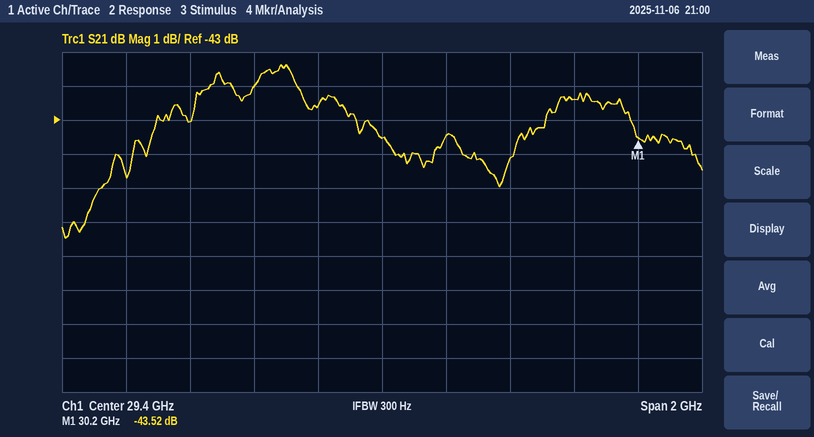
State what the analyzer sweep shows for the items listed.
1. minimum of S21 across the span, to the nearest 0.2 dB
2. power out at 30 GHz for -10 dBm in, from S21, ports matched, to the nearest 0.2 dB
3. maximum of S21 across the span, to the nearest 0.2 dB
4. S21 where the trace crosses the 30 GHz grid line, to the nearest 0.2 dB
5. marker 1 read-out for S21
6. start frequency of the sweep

-46.4 dB
-52.4 dBm
-41.4 dB
-42.4 dB
-43.52 dB
28.4 GHz
